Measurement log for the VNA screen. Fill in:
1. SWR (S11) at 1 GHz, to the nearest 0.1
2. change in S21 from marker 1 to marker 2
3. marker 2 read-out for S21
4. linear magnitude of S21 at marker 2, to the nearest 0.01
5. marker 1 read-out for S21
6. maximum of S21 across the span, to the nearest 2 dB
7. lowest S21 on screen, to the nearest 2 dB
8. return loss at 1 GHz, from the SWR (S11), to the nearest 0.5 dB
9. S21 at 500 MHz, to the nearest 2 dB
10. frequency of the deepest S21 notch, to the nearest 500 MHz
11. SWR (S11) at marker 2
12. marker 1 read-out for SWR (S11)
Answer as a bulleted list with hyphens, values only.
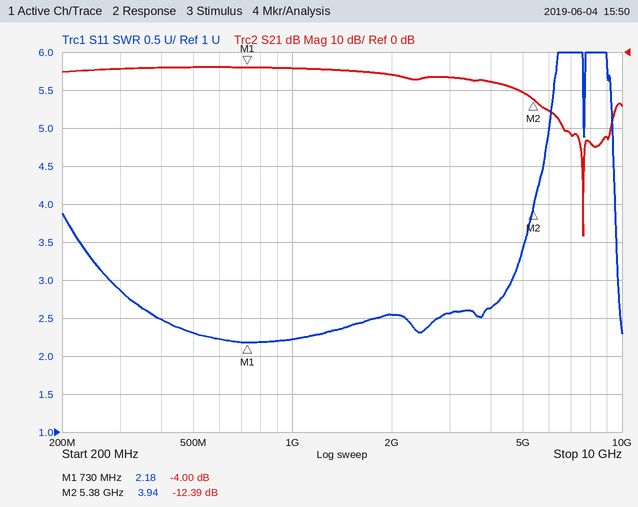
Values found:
- 2.2
- -8.39 dB
- -12.39 dB
- 0.24
- -4.00 dB
- -4 dB
- -48 dB
- 8.5 dB
- -4 dB
- 7.5 GHz
- 3.94
- 2.18
